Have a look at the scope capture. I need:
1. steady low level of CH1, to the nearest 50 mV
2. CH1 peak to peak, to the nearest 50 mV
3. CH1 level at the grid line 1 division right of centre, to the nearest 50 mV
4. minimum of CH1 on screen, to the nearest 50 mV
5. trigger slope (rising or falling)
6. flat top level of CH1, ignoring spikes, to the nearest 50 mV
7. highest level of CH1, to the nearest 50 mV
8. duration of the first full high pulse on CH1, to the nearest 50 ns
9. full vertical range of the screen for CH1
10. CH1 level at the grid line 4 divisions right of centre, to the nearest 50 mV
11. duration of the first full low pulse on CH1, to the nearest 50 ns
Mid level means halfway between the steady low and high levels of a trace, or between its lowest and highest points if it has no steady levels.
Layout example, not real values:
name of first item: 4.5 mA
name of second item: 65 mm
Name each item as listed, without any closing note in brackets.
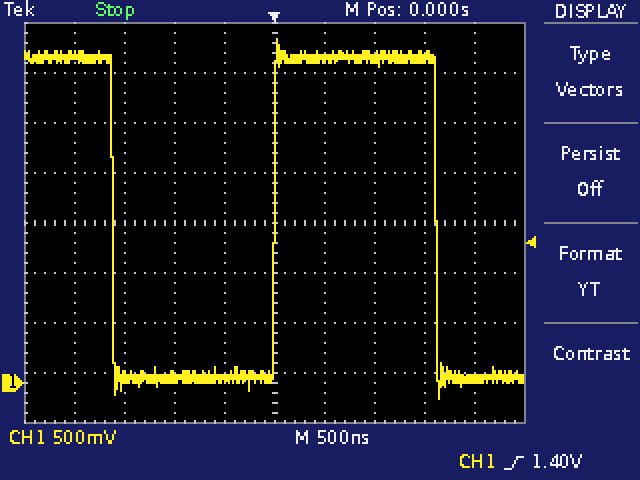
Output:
steady low level of CH1, to the nearest 50 mV: 50 mV
CH1 peak to peak, to the nearest 50 mV: 3.60 V
CH1 level at the grid line 1 division right of centre, to the nearest 50 mV: 3.25 V
minimum of CH1 on screen, to the nearest 50 mV: -150 mV
trigger slope: rising
flat top level of CH1, ignoring spikes, to the nearest 50 mV: 3.25 V
highest level of CH1, to the nearest 50 mV: 3.45 V
duration of the first full high pulse on CH1, to the nearest 50 ns: 1.60 µs
full vertical range of the screen for CH1: 4 V
CH1 level at the grid line 4 divisions right of centre, to the nearest 50 mV: 50 mV
duration of the first full low pulse on CH1, to the nearest 50 ns: 1.60 µs
